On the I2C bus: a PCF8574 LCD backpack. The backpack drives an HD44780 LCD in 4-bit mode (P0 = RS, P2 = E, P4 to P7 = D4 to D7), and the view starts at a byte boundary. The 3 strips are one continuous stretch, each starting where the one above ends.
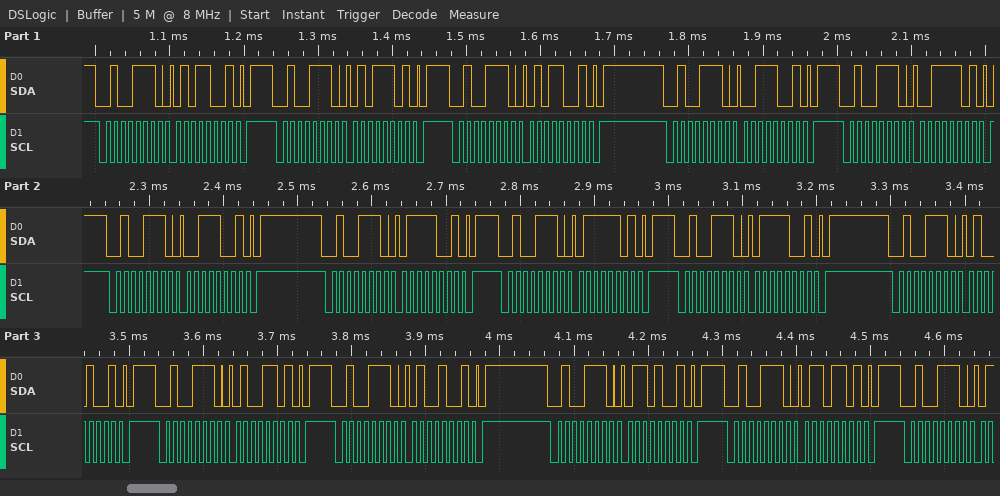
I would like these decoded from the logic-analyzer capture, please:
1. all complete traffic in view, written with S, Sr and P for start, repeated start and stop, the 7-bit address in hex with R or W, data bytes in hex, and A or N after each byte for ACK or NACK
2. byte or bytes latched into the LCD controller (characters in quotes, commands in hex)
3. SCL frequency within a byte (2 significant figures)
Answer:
S 27W A 59 A P S 27W A 5D A P S 27W A 59 A P S 27W A 39 A P S 27W A 3D A P S 27W A 39 A P S 27W A 79 A P S 27W A 7D A P S 27W A 79 A P S 27W A 49 A P S 27W A 4D A P S 27W A 49 A P S 27W A 69 A P S 27W A 6D A P S 27W A
'S' 't'
100 kHz
